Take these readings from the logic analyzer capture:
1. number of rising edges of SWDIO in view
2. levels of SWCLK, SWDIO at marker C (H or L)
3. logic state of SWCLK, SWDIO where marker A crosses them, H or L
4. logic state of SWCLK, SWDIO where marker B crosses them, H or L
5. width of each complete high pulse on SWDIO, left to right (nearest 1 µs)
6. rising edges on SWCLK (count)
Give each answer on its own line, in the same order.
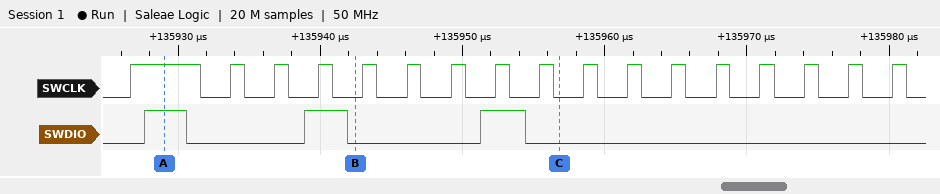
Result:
3
SWCLK=L, SWDIO=L
SWCLK=H, SWDIO=H
SWCLK=L, SWDIO=L
3 µs, 3 µs, 3 µs
17
